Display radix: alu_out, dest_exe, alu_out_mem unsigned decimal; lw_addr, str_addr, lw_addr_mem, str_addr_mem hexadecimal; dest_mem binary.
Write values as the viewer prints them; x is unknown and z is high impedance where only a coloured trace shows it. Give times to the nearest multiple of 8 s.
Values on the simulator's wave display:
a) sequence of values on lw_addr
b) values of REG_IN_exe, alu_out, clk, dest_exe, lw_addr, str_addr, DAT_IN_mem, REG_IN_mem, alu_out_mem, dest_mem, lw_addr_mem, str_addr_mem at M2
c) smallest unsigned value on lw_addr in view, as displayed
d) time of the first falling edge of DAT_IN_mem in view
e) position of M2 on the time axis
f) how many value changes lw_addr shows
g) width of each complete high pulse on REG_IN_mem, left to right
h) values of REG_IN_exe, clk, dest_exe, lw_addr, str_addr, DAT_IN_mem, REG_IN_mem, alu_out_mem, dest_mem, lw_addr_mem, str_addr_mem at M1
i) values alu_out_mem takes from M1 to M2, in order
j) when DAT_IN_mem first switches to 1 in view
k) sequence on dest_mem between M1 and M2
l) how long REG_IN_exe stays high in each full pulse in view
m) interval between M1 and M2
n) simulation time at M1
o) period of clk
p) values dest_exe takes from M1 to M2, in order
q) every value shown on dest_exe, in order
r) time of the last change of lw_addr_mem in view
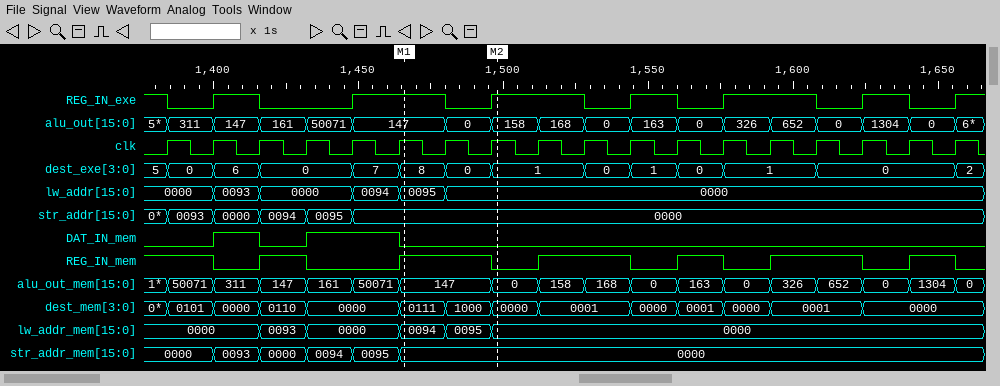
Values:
0000, 0093, 0000, 0094, 0095, 0000
REG_IN_exe=1, alu_out=158, clk=1, dest_exe=1, lw_addr=0000, str_addr=0000, DAT_IN_mem=0, REG_IN_mem=0, alu_out_mem=0, dest_mem=0000, lw_addr_mem=0000, str_addr_mem=0000
0000
1416 s
1496 s
5
16 s, 32 s, 32 s, 16 s, 32 s, 16 s
REG_IN_exe=1, clk=1, dest_exe=8, lw_addr=0095, str_addr=0000, DAT_IN_mem=0, REG_IN_mem=1, alu_out_mem=147, dest_mem=0111, lw_addr_mem=0094, str_addr_mem=0000
147, 0
1400 s
0111, 1000, 0000
16 s, 32 s, 32 s, 16 s, 32 s, 16 s
32 s
1464 s
16 s
8, 0, 1
5, 0, 6, 0, 7, 8, 0, 1, 0, 1, 0, 1, 0, 2
1496 s
